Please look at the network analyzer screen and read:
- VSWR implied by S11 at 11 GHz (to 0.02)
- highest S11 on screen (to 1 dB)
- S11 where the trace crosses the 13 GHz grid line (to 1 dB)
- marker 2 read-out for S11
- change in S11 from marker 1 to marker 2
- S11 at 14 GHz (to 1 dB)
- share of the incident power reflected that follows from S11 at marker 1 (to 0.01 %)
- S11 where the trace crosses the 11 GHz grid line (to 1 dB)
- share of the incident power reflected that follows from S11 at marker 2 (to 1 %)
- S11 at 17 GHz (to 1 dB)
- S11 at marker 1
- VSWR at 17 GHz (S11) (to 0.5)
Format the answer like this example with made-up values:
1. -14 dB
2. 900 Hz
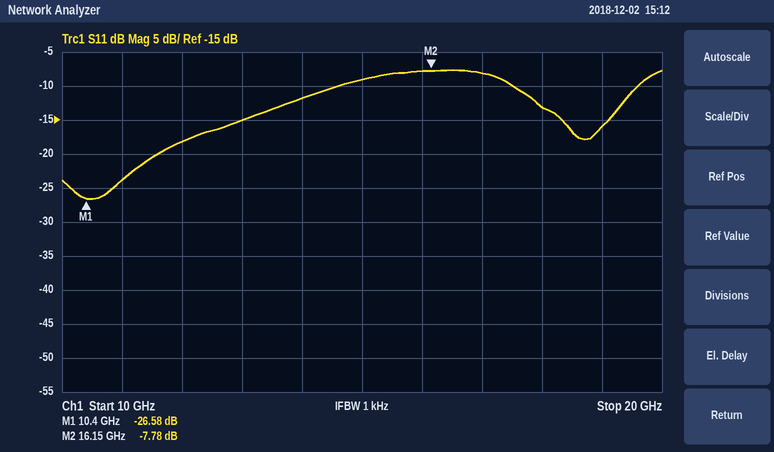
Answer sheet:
1. 1.14
2. -8 dB
3. -15 dB
4. -7.78 dB
5. 18.80 dB
6. -12 dB
7. 0.22 %
8. -24 dB
9. 17 %
10. -8 dB
11. -26.58 dB
12. 2.5
